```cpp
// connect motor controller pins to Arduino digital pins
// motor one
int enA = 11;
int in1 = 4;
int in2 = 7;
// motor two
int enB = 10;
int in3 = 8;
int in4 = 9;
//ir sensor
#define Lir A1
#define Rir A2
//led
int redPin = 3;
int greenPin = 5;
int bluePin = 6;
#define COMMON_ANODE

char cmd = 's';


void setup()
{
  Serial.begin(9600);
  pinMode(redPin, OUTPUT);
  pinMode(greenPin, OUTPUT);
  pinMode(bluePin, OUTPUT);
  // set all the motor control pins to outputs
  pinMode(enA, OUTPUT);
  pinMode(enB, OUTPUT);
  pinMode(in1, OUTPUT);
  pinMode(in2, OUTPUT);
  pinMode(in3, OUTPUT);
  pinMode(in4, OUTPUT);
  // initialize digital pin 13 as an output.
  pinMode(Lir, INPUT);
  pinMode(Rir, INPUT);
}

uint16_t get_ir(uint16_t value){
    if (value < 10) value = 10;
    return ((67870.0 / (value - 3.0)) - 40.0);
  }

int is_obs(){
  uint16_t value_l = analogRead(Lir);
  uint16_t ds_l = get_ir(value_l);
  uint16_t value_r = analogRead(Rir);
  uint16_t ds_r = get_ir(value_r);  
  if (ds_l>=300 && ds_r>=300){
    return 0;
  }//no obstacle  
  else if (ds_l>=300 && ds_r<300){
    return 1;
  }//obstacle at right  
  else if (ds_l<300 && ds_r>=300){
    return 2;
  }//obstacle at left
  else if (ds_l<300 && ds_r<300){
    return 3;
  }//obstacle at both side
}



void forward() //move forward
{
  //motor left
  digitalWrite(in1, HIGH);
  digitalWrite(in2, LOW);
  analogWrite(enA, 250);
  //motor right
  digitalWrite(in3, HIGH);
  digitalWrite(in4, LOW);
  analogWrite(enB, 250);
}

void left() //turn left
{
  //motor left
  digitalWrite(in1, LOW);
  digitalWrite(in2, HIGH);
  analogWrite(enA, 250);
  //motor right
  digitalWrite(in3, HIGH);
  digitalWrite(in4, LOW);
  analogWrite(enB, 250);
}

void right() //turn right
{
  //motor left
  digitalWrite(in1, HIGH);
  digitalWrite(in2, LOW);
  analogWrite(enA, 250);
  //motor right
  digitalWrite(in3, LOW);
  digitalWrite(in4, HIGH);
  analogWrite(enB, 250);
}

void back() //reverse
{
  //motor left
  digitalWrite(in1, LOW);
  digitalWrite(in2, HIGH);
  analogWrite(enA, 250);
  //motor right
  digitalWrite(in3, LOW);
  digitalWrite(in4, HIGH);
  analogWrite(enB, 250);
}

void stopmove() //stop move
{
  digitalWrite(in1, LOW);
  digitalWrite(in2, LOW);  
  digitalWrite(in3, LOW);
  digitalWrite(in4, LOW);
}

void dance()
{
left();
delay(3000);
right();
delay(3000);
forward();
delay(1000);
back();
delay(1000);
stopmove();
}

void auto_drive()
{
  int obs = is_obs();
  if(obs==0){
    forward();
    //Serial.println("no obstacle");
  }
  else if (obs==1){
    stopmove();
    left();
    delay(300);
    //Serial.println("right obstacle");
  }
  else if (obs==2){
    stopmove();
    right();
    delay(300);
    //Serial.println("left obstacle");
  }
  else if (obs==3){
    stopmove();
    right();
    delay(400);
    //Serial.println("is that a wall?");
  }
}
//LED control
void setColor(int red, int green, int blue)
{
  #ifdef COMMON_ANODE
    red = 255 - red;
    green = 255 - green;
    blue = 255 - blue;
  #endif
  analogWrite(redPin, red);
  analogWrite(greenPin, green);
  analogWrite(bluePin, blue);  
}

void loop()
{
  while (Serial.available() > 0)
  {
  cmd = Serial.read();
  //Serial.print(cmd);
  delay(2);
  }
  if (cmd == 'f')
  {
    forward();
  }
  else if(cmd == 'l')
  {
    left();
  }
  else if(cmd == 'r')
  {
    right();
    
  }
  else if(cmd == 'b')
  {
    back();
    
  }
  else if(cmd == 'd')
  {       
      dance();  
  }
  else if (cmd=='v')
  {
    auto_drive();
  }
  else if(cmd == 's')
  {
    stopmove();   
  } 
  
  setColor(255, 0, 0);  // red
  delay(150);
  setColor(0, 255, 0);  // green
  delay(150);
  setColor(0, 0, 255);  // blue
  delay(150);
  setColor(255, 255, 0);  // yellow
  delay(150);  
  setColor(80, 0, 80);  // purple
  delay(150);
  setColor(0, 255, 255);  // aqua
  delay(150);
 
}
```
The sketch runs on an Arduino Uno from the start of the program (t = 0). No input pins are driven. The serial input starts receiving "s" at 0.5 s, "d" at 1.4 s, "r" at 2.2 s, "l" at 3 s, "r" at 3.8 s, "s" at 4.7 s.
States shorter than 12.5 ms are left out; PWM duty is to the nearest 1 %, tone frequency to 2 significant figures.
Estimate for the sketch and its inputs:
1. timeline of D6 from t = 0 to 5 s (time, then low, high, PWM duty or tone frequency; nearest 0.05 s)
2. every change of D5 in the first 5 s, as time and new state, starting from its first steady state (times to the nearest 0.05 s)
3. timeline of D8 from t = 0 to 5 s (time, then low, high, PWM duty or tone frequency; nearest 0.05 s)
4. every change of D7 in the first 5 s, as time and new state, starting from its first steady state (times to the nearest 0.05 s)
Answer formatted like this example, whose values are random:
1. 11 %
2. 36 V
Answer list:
1. 0 s high; 0.3 s low; 0.45 s high; 0.6 s PWM 69 %; 0.75 s low; 0.9 s high; 1.2 s low; 1.35 s high; 1.5 s PWM 69 %; 1.65 s low
2. 0 s high; 0.15 s low; 0.3 s high; 0.45 s low; 0.6 s high; 0.75 s low; 0.9 s high; 1.05 s low; 1.2 s high; 1.35 s low; 1.5 s high; 1.65 s low
3. 0 s low; 1.8 s high; 4.8 s low
4. 0 s low; 1.8 s high; 4.8 s low
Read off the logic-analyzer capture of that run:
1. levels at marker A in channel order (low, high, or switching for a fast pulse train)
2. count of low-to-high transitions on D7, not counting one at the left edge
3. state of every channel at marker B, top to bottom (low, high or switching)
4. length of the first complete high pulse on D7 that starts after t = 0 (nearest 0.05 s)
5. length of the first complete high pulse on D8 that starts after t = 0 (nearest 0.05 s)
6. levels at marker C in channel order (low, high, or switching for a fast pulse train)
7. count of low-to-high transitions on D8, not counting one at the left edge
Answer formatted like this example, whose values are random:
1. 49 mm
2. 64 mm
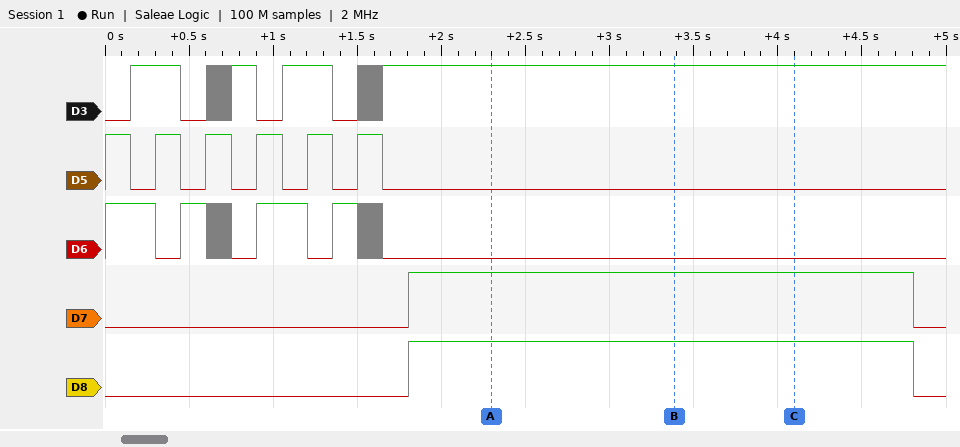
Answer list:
1. D3 high, D5 low, D6 low, D7 high, D8 high
2. 1
3. D3 high, D5 low, D6 low, D7 high, D8 high
4. 3.00 s
5. 3.00 s
6. D3 high, D5 low, D6 low, D7 high, D8 high
7. 1
